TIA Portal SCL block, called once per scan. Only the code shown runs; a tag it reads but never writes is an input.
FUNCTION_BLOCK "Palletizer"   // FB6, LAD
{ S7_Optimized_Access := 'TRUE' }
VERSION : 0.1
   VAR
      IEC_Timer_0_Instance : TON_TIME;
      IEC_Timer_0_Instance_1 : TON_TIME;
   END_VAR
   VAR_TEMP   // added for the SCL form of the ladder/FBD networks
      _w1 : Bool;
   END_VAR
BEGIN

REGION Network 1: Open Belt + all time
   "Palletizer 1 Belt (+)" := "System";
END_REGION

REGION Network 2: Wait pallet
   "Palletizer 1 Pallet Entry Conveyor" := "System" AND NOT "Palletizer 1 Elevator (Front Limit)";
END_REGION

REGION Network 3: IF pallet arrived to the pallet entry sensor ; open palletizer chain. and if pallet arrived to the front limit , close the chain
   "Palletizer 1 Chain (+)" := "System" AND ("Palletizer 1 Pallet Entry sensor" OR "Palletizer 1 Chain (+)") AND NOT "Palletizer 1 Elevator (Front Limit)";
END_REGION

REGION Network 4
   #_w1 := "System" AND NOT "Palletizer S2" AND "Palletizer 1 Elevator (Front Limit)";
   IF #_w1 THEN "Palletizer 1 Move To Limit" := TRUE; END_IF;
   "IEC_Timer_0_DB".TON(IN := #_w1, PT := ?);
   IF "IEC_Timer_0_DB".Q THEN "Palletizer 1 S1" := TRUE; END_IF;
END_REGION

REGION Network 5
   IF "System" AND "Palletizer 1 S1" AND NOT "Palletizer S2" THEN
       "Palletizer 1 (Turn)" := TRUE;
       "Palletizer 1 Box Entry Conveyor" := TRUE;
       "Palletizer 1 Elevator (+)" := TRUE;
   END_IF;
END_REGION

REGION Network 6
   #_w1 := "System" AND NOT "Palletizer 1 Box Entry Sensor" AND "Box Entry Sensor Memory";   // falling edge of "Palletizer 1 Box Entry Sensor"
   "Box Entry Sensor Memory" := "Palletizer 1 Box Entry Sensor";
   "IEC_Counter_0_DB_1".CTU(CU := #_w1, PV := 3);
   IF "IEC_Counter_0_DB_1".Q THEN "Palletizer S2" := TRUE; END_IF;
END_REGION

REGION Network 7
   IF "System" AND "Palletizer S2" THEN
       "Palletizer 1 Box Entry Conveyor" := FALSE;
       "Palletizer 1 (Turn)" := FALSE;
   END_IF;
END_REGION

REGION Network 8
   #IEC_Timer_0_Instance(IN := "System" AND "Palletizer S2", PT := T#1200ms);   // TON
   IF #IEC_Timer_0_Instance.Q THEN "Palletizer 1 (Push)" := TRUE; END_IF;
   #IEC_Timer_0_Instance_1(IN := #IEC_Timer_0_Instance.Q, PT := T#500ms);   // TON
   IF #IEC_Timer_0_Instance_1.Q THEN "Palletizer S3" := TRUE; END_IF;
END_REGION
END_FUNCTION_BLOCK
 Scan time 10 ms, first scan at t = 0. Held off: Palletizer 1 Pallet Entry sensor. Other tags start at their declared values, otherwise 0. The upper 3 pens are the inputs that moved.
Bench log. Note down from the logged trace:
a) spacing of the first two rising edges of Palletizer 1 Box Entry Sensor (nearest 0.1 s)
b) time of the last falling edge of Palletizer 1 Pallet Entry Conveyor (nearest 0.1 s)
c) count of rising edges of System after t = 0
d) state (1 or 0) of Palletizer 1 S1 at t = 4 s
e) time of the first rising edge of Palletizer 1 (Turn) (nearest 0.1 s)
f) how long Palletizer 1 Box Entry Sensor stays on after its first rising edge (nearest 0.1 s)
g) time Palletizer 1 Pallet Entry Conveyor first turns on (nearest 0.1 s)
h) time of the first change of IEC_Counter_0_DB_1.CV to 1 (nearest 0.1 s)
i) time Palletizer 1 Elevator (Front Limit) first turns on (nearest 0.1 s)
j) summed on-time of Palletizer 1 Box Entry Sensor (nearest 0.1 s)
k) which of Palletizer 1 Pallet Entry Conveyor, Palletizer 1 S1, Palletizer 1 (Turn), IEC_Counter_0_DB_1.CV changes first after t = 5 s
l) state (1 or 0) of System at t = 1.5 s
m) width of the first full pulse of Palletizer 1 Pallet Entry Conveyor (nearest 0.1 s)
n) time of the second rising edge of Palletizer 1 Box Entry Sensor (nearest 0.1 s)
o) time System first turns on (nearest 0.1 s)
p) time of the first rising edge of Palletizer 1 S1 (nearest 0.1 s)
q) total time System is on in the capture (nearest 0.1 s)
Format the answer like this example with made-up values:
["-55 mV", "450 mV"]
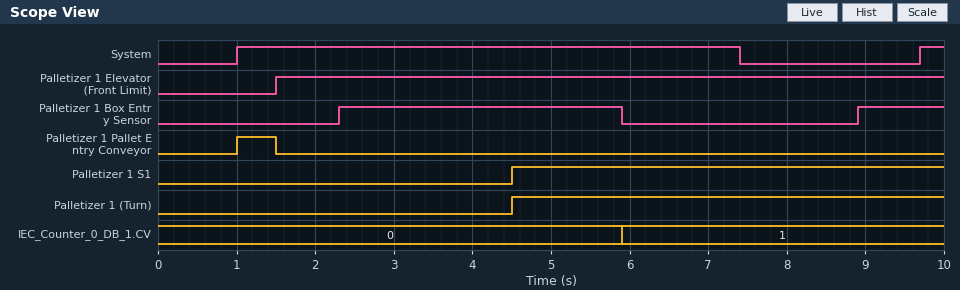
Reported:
["6.6 s", "1.5 s", "2", "0", "4.5 s", "3.6 s", "1.0 s", "5.9 s", "1.5 s", "4.7 s", "IEC_Counter_0_DB_1.CV", "1", "0.5 s", "8.9 s", "1.0 s", "4.5 s", "6.7 s"]
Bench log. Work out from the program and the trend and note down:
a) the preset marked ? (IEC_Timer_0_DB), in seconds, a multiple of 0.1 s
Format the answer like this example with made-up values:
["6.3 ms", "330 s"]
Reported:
["3.0 s"]
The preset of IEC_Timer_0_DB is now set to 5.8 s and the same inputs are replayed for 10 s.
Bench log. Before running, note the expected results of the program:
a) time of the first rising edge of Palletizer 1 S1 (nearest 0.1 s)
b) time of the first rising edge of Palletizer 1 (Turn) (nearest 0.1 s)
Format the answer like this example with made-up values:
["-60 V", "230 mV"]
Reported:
["7.3 s", "7.3 s"]
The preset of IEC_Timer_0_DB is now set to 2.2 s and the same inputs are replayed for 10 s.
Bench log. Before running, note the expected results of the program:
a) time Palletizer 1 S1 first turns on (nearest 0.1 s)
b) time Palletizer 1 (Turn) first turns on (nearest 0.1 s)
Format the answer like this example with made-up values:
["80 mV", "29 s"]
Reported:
["3.7 s", "3.7 s"]
